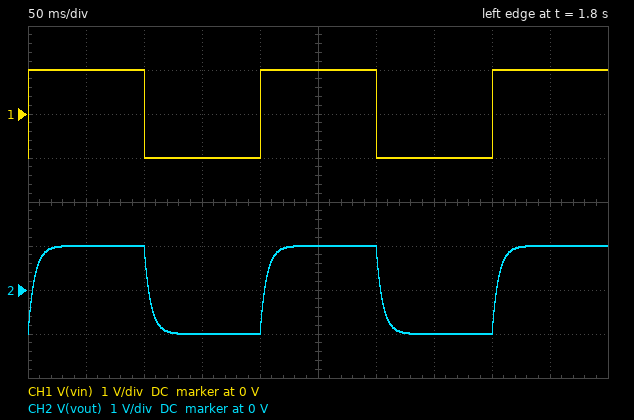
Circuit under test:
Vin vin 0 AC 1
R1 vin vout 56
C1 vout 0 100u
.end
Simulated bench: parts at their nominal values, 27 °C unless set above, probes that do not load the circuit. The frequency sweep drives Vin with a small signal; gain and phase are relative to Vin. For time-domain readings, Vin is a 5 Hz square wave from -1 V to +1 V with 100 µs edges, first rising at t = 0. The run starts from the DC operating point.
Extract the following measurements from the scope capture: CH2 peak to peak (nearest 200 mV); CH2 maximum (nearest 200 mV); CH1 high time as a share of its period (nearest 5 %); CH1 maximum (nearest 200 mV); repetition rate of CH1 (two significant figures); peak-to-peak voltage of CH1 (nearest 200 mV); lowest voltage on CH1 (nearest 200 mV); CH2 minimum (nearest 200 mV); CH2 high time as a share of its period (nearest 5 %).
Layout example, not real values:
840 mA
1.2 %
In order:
2.0 V
1.0 V
50 %
1.0 V
5.0 Hz
2.0 V
-1.0 V
-1.0 V
50 %
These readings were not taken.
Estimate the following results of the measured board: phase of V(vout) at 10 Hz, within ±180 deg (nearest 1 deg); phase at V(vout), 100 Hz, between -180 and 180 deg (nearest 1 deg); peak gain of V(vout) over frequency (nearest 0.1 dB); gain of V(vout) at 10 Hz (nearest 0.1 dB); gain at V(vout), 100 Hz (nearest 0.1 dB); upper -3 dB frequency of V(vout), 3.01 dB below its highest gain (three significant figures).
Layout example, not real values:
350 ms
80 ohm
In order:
-19 deg
-74 deg
0 dB
-0.5 dB
-11.3 dB
28.4 Hz
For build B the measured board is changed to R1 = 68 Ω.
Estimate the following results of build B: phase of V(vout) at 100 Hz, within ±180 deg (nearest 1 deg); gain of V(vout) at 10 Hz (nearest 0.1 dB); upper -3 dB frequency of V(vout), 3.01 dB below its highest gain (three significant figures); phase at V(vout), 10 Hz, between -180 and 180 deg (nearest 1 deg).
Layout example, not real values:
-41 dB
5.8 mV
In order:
-77 deg
-0.7 dB
23.4 Hz
-23 deg
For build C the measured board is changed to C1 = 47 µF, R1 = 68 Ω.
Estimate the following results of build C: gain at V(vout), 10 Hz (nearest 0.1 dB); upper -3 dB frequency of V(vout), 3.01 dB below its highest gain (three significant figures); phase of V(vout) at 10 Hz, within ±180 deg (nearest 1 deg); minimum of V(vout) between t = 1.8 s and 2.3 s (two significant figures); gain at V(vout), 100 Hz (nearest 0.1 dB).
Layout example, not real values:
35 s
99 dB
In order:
-0.2 dB
49.8 Hz
-11 deg
-1.0 V
-7.0 dB
